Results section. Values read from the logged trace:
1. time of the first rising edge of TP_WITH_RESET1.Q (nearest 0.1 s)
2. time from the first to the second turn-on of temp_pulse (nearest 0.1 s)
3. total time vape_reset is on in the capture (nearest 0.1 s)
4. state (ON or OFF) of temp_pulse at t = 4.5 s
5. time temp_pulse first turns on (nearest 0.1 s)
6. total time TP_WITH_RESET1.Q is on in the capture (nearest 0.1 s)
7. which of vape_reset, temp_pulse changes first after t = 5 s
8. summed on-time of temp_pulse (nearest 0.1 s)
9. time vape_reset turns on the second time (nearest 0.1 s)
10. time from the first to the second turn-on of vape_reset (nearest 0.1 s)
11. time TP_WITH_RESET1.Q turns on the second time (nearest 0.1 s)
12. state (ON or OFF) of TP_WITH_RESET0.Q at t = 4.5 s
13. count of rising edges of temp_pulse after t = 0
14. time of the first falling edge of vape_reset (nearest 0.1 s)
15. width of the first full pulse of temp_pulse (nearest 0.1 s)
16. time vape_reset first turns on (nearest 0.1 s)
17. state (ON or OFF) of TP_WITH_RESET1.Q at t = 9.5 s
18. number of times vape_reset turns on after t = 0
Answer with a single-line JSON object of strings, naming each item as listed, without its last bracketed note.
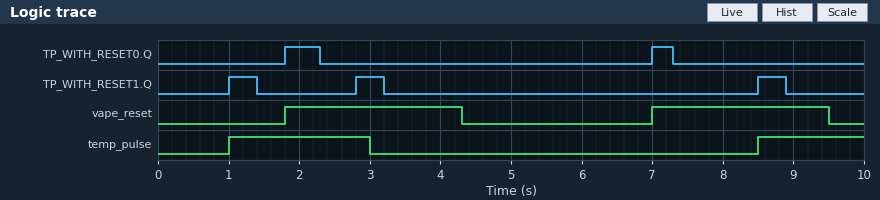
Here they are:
{"time of the first rising edge of TP_WITH_RESET1.Q": "1.0 s", "time from the first to the second turn-on of temp_pulse": "7.5 s", "total time vape_reset is on in the capture": "5.0 s", "state (ON or OFF) of temp_pulse at t = 4.5 s": "OFF", "time temp_pulse first turns on": "1.0 s", "total time TP_WITH_RESET1.Q is on in the capture": "1.2 s", "which of vape_reset, temp_pulse changes first after t = 5 s": "vape_reset", "summed on-time of temp_pulse": "3.5 s", "time vape_reset turns on the second time": "7.0 s", "time from the first to the second turn-on of vape_reset": "5.2 s", "time TP_WITH_RESET1.Q turns on the second time": "2.8 s", "state (ON or OFF) of TP_WITH_RESET0.Q at t = 4.5 s": "OFF", "count of rising edges of temp_pulse after t = 0": "2", "time of the first falling edge of vape_reset": "4.3 s", "width of the first full pulse of temp_pulse": "2.0 s", "time vape_reset first turns on": "1.8 s", "state (ON or OFF) of TP_WITH_RESET1.Q at t = 9.5 s": "OFF", "number of times vape_reset turns on after t = 0": "2"}
